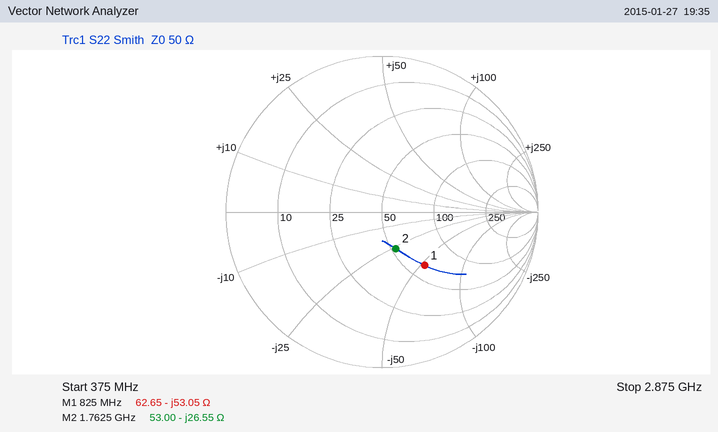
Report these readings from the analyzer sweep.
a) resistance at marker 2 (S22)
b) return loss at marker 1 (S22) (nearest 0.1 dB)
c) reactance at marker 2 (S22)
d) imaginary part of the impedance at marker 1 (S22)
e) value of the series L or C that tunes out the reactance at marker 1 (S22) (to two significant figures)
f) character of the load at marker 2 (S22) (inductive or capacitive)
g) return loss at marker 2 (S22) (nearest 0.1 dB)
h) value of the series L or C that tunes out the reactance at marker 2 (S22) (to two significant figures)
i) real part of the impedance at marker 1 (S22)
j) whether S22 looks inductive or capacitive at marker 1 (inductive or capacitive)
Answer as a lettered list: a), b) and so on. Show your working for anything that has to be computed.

a) 53.00 Ω
b) 7.2 dB
c) -26.55 Ω
d) -53.05 Ω
e) L = 53.05 Ω/(2π × 825 MHz) ≈ 10 nH
f) capacitive
g) 12.0 dB
h) L = 26.55 Ω/(2π × 1.7625 GHz) ≈ 2.4 nH
i) 62.65 Ω
j) capacitive
